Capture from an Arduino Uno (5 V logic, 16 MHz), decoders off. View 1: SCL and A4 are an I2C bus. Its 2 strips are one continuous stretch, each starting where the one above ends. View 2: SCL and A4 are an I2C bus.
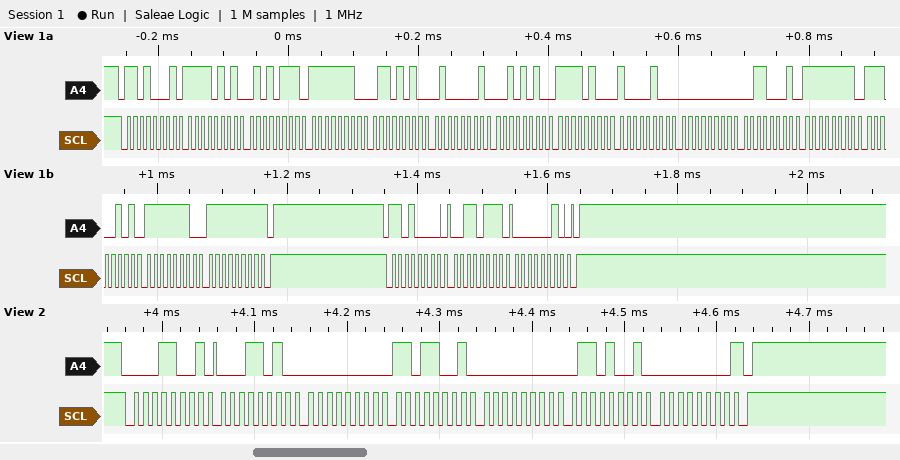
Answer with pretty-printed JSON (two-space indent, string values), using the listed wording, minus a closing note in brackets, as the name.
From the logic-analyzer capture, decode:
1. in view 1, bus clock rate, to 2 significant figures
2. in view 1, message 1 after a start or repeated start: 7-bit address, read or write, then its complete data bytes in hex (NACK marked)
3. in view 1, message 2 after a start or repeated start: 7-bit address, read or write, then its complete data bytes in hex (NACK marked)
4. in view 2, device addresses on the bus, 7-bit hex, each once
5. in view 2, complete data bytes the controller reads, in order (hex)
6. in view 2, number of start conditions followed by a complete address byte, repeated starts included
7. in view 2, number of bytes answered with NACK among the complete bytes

{
  "in view 1, bus clock rate, to 2 significant figures": "100 kHz",
  "in view 1, message 1 after a start or repeated start: 7-bit address, read or write, then its complete data bytes in hex": "0x68 read: F5 57 FE 6A 41 2A F4 84 00 31 FF E5 FE FF NACK",
  "in view 1, message 2 after a start or repeated start: 7-bit address, read or write, then its complete data bytes in hex": "0x68 write: 37 02",
  "in view 2, device addresses on the bus, 7-bit hex, each once": "0x0C",
  "in view 2, complete data bytes the controller reads, in order": "1A 00 D9 00 69 00",
  "in view 2, number of start conditions followed by a complete address byte, repeated starts included": "1",
  "in view 2, number of bytes answered with NACK among the complete bytes": "1"
}
